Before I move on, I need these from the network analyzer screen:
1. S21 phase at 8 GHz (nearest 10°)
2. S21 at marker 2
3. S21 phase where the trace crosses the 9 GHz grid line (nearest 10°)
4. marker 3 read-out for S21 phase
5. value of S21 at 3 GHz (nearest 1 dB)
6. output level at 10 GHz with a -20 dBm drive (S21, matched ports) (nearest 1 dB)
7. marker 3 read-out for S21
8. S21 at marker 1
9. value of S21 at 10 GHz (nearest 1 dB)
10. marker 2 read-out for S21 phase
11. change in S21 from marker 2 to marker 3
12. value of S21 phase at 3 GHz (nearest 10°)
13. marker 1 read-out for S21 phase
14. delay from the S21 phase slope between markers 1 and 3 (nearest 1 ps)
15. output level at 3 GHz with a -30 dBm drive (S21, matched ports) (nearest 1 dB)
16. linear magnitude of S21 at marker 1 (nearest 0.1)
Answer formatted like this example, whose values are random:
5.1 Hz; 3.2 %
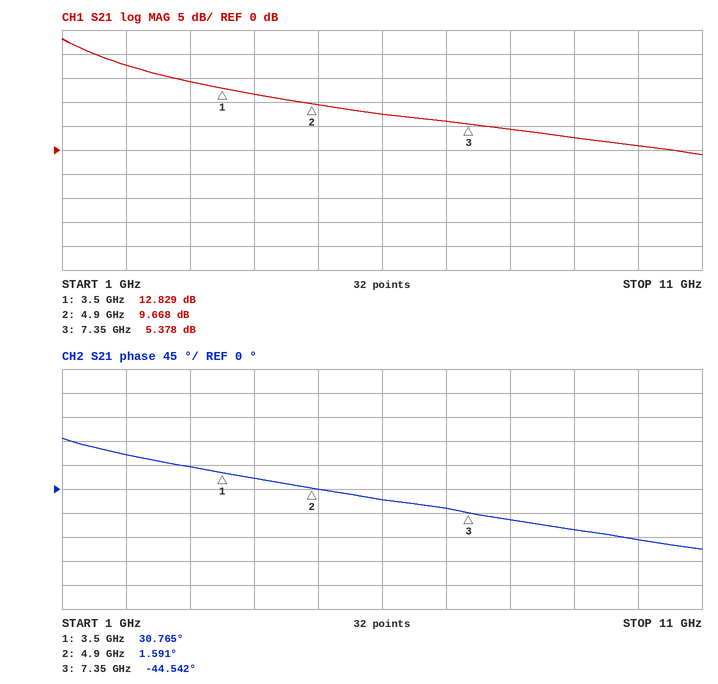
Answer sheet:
-60°; 9.668 dB; -80°; -44.542°; 14 dB; -19 dBm; 5.378 dB; 12.829 dB; 1 dB; 1.591°; -4.290 dB; 40°; 30.765°; 54 ps; -16 dBm; 4.4
